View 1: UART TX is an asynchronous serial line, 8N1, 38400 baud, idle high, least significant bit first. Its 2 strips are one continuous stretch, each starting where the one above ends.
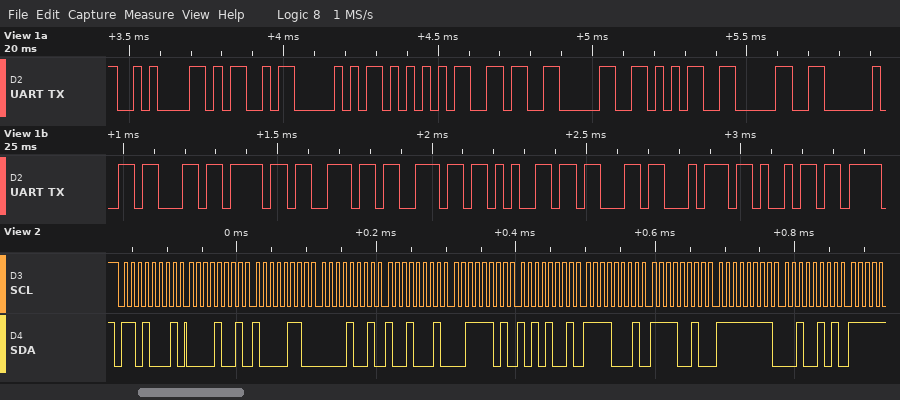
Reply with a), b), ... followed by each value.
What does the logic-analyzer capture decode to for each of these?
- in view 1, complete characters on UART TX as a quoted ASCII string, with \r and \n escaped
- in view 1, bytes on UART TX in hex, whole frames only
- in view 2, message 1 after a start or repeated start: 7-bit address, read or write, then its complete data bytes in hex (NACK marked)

a) "\nMPU6050 connecti"
b) 0A 4D 50 55 36 30 35 30 20 63 6F 6E 6E 65 63 74 69
c) 0x68 read: 09 86 09 91 3D A9 F1 F2 FF 25
